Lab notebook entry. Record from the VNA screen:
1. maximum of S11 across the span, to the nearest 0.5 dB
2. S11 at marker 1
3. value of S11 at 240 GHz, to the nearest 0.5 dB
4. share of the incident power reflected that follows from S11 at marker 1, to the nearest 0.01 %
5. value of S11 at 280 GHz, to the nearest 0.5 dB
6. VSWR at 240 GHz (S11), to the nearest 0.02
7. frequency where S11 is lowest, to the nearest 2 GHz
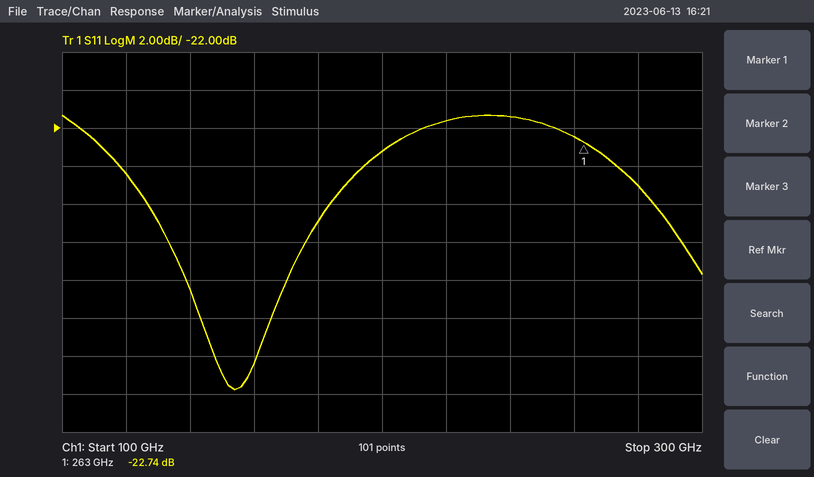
-21.5 dB
-22.74 dB
-21.5 dB
0.53 %
-25.0 dB
1.18
154 GHz
